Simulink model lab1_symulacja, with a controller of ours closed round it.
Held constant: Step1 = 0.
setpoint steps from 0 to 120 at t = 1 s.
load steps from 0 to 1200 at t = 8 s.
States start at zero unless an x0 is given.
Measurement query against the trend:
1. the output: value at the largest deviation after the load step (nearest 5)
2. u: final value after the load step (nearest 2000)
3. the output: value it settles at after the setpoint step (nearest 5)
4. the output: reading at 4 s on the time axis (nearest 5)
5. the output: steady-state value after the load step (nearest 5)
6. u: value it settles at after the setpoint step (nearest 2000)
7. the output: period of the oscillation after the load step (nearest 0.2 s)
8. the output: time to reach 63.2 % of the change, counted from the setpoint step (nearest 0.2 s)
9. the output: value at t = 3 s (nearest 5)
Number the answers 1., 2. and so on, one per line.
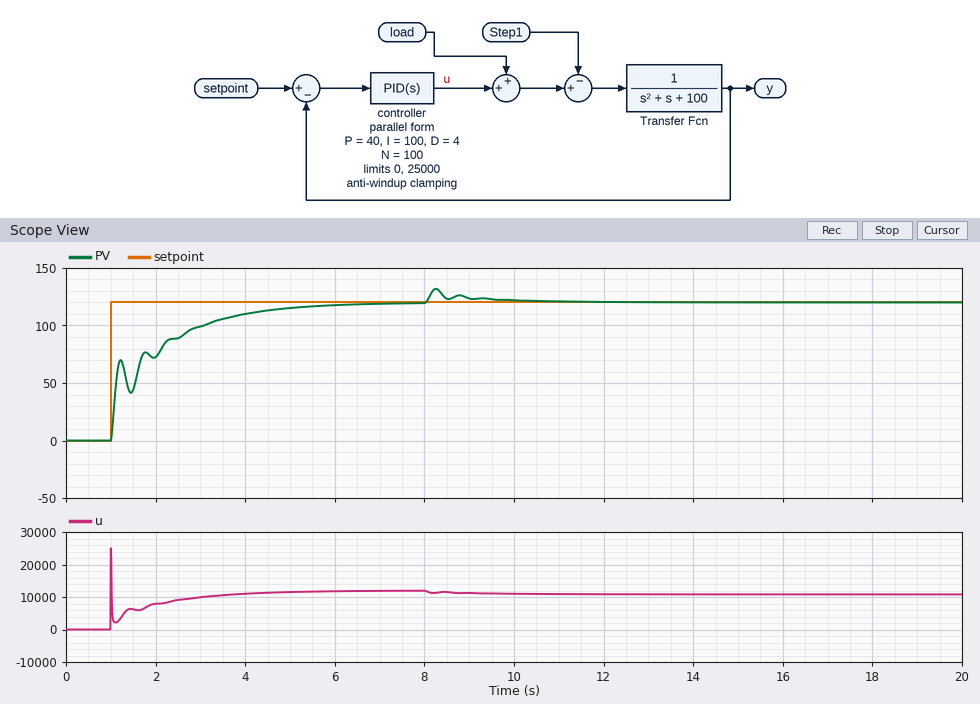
1. 130
2. 10000
3. 120
4. 110
5. 120
6. 12000
7. 0.6 s
8. 0.8 s
9. 100
